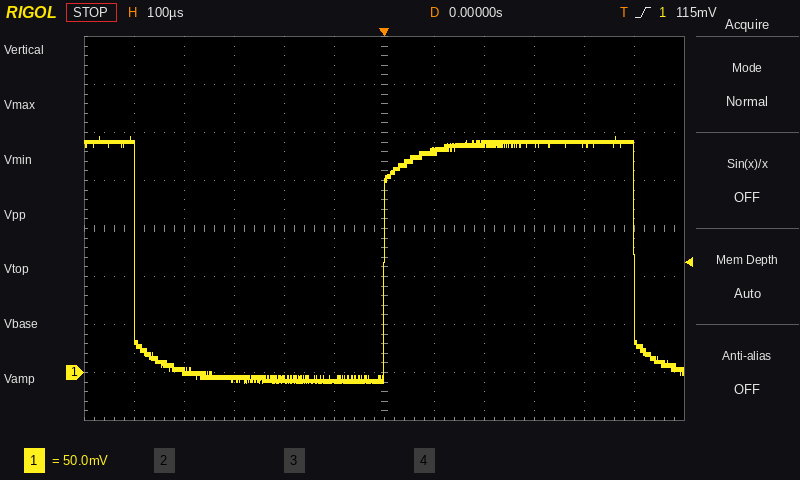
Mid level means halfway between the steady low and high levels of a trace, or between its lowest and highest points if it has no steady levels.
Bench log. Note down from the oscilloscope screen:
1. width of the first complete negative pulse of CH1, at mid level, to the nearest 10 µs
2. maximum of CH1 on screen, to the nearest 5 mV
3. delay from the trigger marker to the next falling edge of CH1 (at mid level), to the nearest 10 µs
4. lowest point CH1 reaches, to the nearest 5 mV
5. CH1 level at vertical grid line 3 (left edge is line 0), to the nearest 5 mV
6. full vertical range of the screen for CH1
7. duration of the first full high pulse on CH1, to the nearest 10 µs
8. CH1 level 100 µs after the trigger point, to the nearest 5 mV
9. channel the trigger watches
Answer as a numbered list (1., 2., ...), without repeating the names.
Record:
1. 500 µs
2. 245 mV
3. 500 µs
4. -10 mV
5. -5 mV
6. 400 mV
7. 500 µs
8. 230 mV
9. CH1
